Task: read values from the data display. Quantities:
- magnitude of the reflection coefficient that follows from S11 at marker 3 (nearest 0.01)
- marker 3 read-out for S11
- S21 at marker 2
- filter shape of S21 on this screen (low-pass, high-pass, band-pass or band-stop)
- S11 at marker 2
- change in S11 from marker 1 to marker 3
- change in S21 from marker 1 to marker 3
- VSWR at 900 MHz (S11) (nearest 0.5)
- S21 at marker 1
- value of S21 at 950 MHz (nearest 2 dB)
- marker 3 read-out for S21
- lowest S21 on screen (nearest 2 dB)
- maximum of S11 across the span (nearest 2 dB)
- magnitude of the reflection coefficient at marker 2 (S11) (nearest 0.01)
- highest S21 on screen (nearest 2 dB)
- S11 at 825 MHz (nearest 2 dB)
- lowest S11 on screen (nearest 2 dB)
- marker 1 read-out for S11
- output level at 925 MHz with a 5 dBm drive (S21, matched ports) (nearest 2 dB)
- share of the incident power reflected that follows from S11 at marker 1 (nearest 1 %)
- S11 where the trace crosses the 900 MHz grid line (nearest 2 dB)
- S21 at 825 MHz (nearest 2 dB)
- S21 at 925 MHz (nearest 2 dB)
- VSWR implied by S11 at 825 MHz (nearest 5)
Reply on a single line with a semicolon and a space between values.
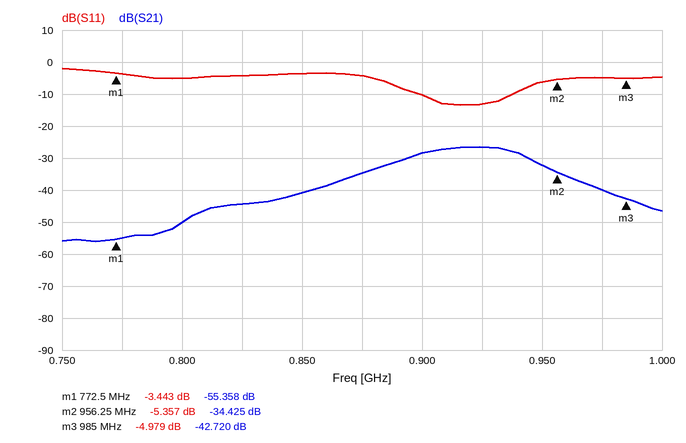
0.56; -4.979 dB; -34.425 dB; band-pass; -5.357 dB; -1.536 dB; 12.638 dB; 2.0; -55.358 dB; -32 dB; -42.720 dB; -56 dB; -2 dB; 0.54; -26 dB; -4 dB; -14 dB; -3.443 dB; -22 dBm; 45 %; -10 dB; -44 dB; -26 dB; 5
